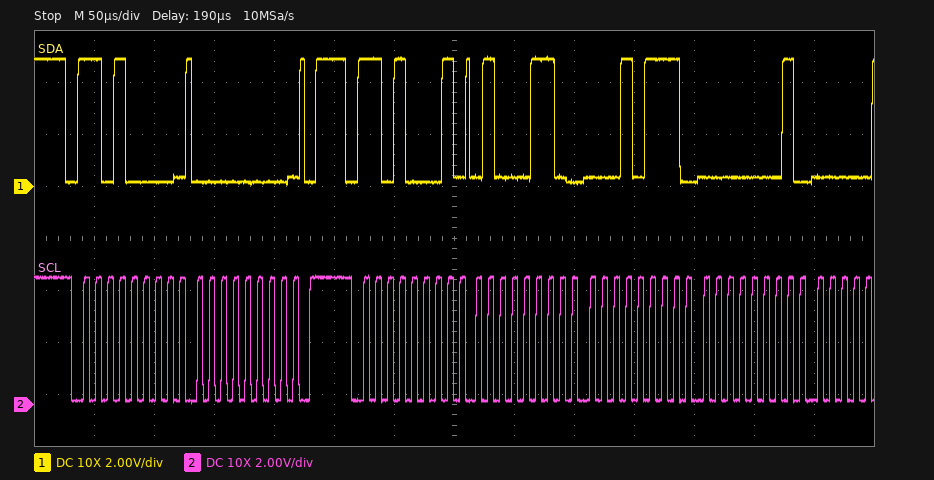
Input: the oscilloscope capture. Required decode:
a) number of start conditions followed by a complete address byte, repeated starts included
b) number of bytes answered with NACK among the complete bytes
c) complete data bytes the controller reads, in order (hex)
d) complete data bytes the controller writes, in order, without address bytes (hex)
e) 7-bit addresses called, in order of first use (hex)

2
0
46 17 01
00
0x68
